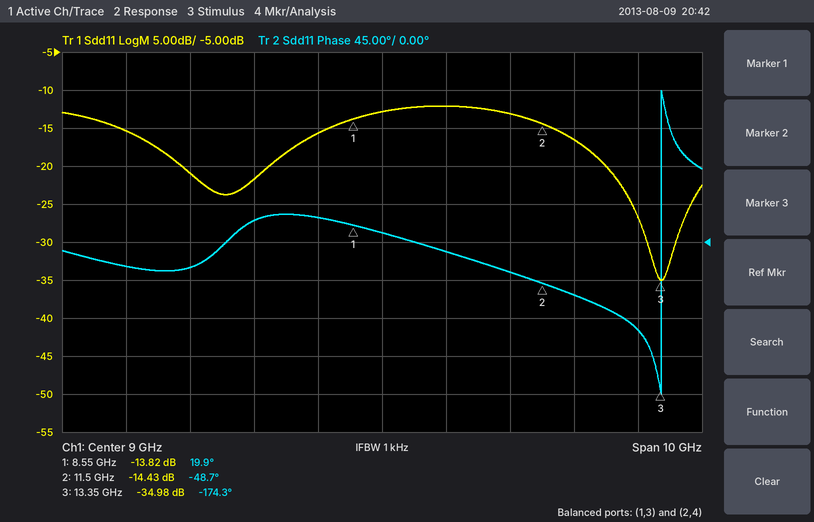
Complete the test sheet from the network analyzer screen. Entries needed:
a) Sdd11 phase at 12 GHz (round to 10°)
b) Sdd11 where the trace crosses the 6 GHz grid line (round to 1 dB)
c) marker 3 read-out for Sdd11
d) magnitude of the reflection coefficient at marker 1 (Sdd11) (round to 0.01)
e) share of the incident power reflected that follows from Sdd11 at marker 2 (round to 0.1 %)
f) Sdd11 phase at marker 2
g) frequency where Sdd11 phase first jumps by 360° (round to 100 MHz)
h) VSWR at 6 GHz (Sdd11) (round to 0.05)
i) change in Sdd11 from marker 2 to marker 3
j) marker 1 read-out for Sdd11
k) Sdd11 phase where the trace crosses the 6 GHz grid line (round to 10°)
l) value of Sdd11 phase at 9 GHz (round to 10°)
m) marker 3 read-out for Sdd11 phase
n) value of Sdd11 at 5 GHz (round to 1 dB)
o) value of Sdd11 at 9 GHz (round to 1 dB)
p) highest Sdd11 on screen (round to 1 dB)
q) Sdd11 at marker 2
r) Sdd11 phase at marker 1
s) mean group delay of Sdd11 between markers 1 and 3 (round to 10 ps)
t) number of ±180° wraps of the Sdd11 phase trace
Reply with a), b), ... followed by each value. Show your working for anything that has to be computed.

a) -60°
b) -21 dB
c) -34.98 dB
d) 10^(-13.82/20) ≈ 0.20
e) 10^(-14.43/10) ≈ 3.6 %
f) -48.7°
g) 13.4 GHz
h) |Γ| = 10^(-21/20) = 0.0891; VSWR = (1 + 0.0891)/(1 − 0.0891) ≈ 1.20
i) -34.98 − (-14.43) = -20.55 dB
j) -13.82 dB
k) -30°
l) 10°
m) -174.3°
n) -15 dB
o) -13 dB
p) -12 dB
q) -14.43 dB
r) 19.9°
s) −(-174.3° − (19.9°))/(360° × 4.8 GHz) ≈ 112 ps, so 110 ps to the nearest 10 ps
t) 1
